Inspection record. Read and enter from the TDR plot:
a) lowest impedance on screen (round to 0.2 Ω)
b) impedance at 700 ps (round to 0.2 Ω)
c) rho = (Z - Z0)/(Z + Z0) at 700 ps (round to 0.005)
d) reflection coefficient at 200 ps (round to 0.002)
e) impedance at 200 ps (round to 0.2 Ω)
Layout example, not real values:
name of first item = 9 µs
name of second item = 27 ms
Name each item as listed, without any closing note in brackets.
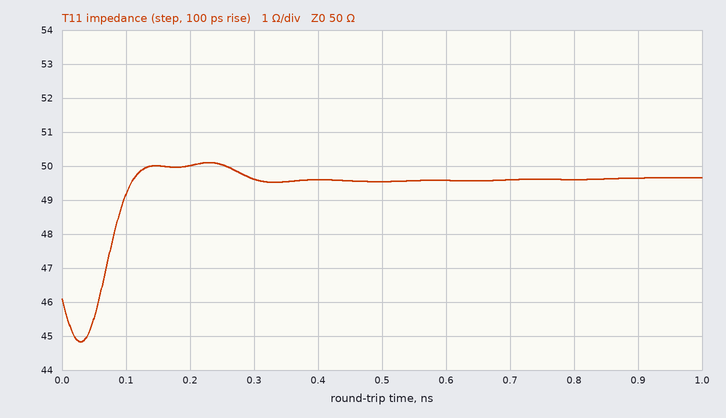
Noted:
lowest impedance on screen = 44.8 Ω
impedance at 700 ps = 49.6 Ω
rho = (Z - Z0)/(Z + Z0) at 700 ps = -0.005
reflection coefficient at 200 ps = 0.000
impedance at 200 ps = 50.0 Ω
